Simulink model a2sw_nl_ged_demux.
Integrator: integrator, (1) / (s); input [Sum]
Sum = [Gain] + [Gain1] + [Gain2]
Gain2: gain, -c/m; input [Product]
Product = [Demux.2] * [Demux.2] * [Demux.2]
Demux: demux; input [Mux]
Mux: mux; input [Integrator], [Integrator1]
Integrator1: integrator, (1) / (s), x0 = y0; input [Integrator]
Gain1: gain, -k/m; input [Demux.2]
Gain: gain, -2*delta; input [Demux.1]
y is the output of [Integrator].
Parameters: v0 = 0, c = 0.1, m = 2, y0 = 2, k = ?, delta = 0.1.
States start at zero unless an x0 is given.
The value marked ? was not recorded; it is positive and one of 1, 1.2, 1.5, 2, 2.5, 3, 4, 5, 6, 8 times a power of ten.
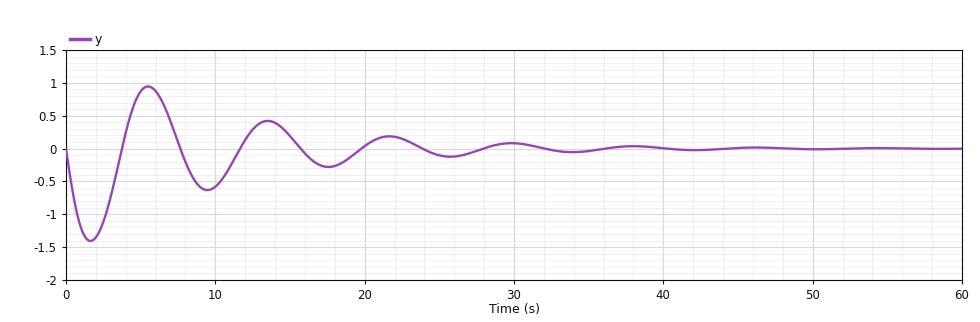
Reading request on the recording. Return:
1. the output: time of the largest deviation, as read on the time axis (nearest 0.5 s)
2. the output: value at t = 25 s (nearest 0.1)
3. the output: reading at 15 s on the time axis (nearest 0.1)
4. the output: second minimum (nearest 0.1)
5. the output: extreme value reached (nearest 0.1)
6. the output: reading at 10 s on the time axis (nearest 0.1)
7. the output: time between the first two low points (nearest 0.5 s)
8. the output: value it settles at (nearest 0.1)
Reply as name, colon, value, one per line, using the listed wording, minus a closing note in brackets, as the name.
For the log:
the output: time of the largest deviation, as read on the time axis: 1.5 s
the output: value at t = 25 s: -0.1
the output: reading at 15 s on the time axis: 0.2
the output: second minimum: -0.6
the output: extreme value reached: -1.4
the output: reading at 10 s on the time axis: -0.6
the output: time between the first two low points: 8.0 s
the output: value it settles at: 0.0
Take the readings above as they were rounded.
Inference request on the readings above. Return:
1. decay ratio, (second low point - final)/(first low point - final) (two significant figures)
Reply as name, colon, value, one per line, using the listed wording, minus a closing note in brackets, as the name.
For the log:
decay ratio, (second low point - final)/(first low point - final): 0.43
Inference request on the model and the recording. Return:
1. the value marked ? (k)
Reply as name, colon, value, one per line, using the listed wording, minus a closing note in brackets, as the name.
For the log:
the value marked ?: 1.2
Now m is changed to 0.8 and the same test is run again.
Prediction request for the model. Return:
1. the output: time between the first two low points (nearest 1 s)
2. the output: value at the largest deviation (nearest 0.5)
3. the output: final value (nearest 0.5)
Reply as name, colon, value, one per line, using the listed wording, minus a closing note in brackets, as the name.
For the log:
the output: time between the first two low points: 5 s
the output: value at the largest deviation: -2.5
the output: final value: 0.0
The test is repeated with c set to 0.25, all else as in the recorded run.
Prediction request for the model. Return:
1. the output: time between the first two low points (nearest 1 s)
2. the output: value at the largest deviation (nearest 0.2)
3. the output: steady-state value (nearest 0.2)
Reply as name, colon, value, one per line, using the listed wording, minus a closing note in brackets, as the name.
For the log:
the output: time between the first two low points: 7 s
the output: value at the largest deviation: -1.6
the output: steady-state value: 0.0
